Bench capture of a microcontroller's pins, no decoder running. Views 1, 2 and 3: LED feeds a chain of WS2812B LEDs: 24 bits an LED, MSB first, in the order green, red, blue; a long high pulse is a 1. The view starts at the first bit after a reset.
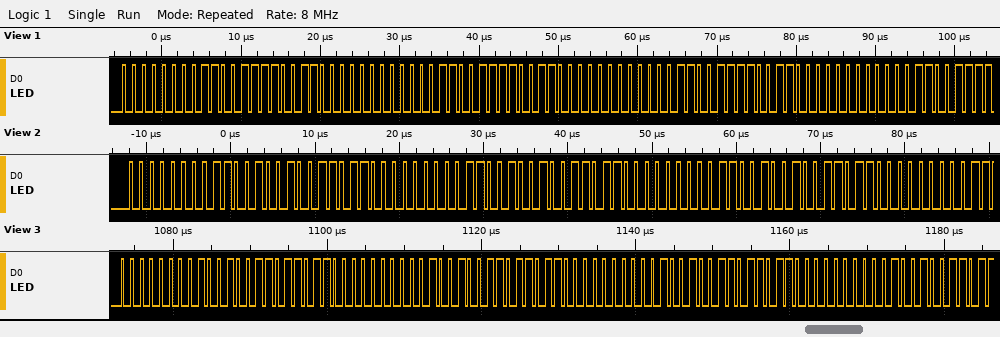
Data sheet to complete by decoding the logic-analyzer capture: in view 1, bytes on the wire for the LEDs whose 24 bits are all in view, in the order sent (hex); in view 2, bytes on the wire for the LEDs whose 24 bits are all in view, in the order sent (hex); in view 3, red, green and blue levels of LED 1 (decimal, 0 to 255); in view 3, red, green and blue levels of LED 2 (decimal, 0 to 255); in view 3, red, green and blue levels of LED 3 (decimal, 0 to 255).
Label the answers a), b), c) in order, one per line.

a) 00 CF 30 00 CF 30 00 CF 30
b) 00 C9 36 00 C9 36 00 C9 36
c) 147, 0, 108
d) 147, 0, 108
e) 147, 0, 108
